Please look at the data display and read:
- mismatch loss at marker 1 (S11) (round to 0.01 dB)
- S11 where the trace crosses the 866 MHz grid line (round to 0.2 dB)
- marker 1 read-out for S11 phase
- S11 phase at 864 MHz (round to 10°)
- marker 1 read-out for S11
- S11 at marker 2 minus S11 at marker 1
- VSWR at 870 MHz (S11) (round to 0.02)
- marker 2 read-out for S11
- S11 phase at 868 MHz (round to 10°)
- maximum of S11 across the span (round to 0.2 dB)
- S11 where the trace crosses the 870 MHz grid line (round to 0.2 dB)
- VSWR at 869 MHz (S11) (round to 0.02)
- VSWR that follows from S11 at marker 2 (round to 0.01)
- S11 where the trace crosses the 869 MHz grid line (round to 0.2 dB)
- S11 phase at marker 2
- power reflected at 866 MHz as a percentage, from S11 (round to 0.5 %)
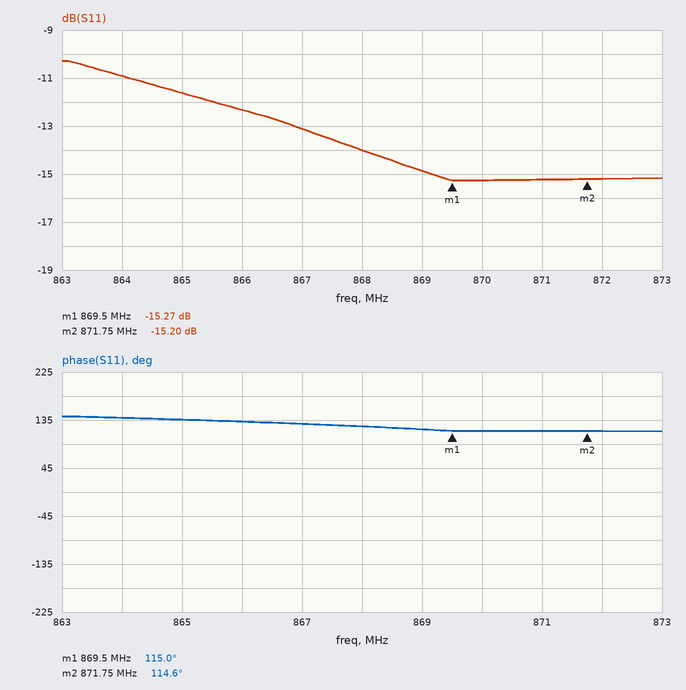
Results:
0.13 dB
-12.4 dB
115.0°
140°
-15.27 dB
0.07 dB
1.42
-15.20 dB
120°
-10.2 dB
-15.2 dB
1.44
1.42
-14.8 dB
114.6°
6.0 %
